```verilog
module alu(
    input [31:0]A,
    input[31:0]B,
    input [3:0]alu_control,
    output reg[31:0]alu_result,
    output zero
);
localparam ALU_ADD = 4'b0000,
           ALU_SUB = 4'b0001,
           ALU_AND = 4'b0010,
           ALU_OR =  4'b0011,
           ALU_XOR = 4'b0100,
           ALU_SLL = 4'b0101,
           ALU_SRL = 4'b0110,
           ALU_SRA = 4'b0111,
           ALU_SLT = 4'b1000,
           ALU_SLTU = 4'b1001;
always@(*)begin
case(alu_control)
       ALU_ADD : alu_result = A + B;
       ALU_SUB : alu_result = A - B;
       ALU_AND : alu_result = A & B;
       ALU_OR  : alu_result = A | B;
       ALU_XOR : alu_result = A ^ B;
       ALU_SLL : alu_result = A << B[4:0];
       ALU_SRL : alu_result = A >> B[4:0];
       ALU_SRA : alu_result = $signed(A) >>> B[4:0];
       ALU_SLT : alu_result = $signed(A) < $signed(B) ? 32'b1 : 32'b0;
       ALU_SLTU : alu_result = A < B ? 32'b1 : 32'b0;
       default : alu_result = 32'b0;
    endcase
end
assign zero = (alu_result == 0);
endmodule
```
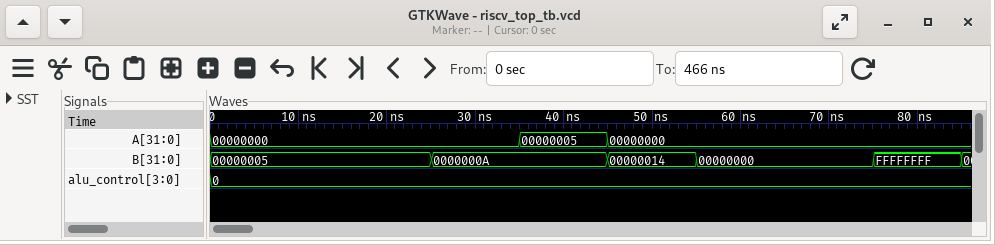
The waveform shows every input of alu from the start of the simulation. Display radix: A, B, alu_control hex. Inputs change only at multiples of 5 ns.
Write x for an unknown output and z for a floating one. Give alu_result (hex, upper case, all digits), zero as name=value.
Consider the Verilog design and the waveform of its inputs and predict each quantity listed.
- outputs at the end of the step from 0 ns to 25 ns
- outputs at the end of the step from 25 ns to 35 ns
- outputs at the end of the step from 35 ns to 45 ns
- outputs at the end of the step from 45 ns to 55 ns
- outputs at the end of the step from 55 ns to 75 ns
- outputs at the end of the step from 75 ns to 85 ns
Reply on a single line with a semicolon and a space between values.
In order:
alu_result=00000005, zero=0; alu_result=0000000A, zero=0; alu_result=0000000F, zero=0; alu_result=00000014, zero=0; alu_result=00000000, zero=1; alu_result=FFFFFFFF, zero=0
